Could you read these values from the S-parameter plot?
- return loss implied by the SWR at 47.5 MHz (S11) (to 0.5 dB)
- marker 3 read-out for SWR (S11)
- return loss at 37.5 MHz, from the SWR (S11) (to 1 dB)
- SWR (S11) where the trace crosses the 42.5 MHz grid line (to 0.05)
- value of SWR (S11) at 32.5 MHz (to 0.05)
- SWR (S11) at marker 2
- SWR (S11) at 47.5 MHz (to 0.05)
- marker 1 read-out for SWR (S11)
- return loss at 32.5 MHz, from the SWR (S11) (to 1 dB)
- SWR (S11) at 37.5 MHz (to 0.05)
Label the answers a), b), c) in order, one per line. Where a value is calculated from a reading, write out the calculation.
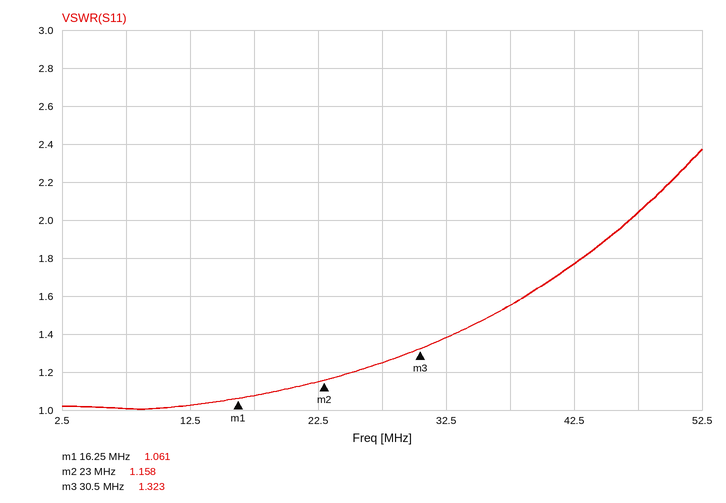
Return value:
a) −20 log10((2.05 − 1)/(2.05 + 1)) ≈ 9.26 dB, so 9.5 dB to the nearest 0.5 dB
b) 1.323
c) −20 log10((1.55 − 1)/(1.55 + 1)) ≈ 13 dB
d) 1.75
e) 1.40
f) 1.158
g) 2.05
h) 1.061
i) −20 log10((1.4 − 1)/(1.4 + 1)) ≈ 16 dB
j) 1.55
